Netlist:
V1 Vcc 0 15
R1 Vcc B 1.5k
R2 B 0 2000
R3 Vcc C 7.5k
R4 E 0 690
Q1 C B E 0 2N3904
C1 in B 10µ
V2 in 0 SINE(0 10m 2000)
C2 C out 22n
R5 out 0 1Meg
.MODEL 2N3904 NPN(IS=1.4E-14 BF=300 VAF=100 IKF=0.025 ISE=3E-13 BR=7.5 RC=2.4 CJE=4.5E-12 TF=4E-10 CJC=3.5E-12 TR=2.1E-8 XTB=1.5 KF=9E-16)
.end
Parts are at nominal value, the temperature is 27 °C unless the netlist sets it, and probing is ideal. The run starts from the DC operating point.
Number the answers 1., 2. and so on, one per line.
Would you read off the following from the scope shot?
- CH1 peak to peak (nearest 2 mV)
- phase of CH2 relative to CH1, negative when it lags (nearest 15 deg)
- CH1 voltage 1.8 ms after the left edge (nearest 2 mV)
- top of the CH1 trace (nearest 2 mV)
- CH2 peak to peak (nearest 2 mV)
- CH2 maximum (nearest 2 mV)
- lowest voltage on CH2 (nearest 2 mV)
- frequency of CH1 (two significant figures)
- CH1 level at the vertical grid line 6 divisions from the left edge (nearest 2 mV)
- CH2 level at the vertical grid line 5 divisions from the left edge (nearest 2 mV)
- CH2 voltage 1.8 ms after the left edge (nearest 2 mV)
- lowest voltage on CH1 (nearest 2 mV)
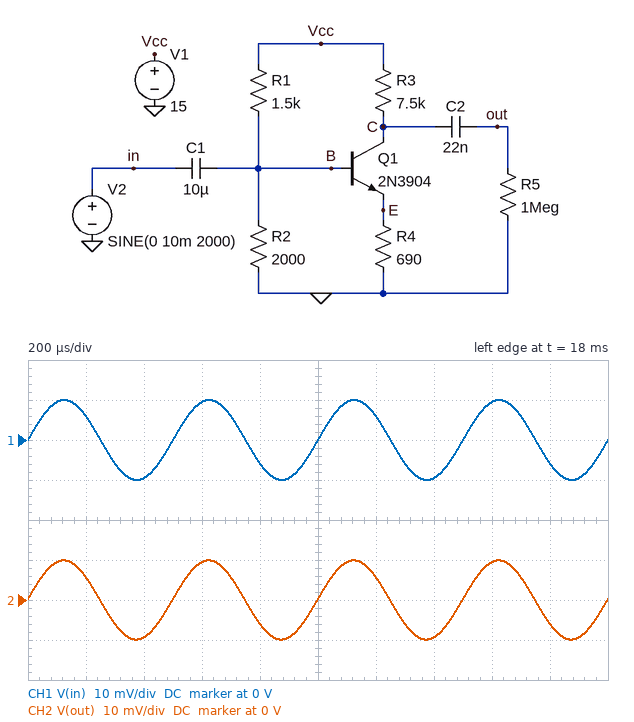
1. 20 mV
2. 0 deg
3. -6 mV
4. 10 mV
5. 20 mV
6. 10 mV
7. -10 mV
8. 2.0 kHz
9. 6 mV
10. 0 V
11. -6 mV
12. -10 mV
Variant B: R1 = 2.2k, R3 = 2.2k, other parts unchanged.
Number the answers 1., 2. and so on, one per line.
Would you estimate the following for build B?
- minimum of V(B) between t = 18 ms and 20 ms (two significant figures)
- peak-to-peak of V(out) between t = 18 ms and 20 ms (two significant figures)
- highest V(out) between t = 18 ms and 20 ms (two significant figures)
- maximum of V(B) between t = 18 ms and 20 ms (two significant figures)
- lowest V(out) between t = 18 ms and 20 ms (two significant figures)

1. 5.2 V
2. 19 mV
3. 9.7 mV
4. 5.3 V
5. -9.7 mV
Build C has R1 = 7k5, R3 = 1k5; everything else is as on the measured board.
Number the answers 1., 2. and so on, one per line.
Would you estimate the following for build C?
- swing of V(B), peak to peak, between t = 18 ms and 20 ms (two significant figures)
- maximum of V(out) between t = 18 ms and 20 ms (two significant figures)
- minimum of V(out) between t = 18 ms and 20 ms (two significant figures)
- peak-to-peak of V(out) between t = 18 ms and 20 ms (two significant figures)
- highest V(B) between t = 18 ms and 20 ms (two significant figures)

1. 20 mV
2. 21 mV
3. -21 mV
4. 43 mV
5. 3.1 V
